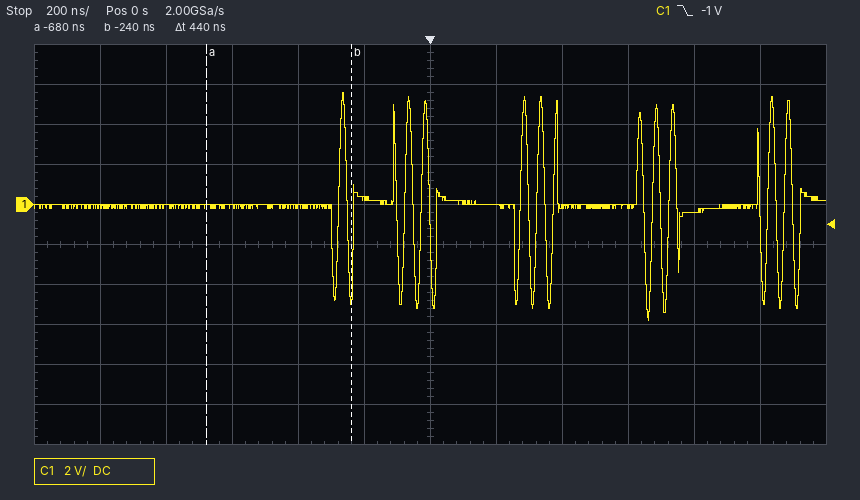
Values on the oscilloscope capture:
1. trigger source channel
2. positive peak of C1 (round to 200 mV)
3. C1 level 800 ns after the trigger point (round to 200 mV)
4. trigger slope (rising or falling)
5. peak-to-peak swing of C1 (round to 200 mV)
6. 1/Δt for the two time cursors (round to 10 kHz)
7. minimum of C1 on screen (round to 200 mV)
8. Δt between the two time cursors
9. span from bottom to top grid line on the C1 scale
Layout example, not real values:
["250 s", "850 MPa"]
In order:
["C1", "5.6 V", "-400 mV", "falling", "11.4 V", "2.27 MHz", "-5.8 V", "440 ns", "20 V"]
